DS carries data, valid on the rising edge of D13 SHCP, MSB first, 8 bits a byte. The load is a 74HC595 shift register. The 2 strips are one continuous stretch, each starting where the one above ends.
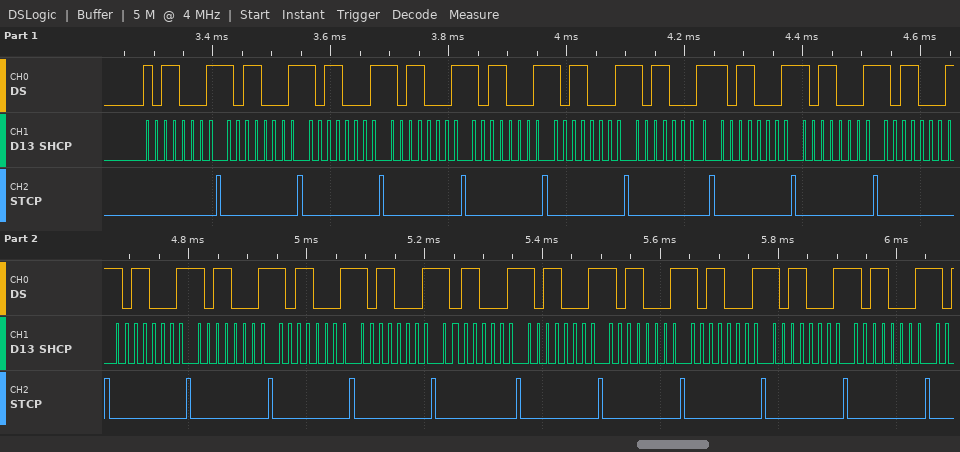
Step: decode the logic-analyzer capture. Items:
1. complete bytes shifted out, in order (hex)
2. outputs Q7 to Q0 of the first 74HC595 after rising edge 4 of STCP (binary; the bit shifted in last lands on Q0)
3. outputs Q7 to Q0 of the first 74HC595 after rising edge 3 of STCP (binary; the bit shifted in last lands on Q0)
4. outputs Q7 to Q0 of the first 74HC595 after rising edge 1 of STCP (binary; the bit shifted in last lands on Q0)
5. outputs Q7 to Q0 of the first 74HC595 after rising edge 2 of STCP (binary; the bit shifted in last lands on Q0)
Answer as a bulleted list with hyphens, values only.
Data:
- B1 B1 B1 B1 B1 B1 B1 B1 B1 B1 B1 B1 B1 B1 B1 B1 B1 B1 B1 B1
- 10110001
- 10110001
- 10110001
- 10110001
